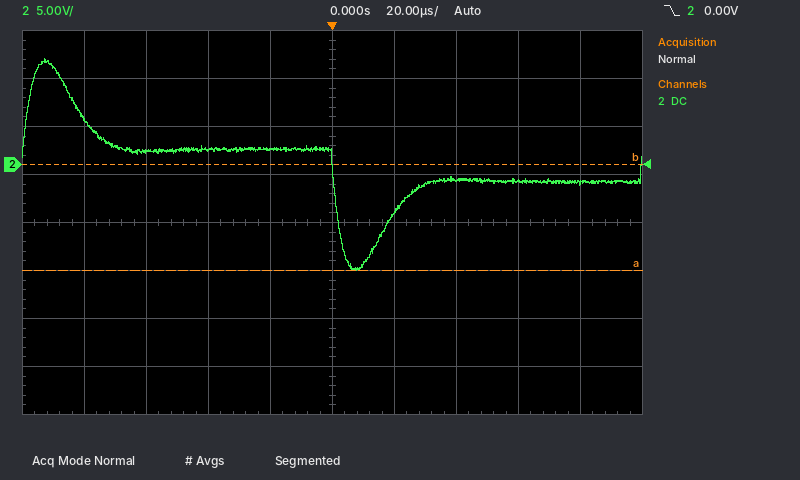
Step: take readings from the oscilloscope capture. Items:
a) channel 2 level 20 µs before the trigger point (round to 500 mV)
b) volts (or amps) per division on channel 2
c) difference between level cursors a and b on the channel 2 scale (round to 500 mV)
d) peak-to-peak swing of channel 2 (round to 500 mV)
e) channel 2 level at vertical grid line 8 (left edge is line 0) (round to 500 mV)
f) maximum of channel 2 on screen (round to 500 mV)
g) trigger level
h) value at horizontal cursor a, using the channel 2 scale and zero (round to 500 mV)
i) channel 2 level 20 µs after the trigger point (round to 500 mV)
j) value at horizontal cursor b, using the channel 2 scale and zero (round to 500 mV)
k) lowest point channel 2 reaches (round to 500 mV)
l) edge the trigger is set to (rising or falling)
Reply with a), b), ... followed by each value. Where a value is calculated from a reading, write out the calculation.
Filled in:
a) 1.5 V
b) 5 V
c) 11.0 V
d) 11.0 V − (-11.0 V) = 22.0 V
e) -1.5 V
f) 11.0 V
g) 0.00 V
h) -11.0 V
i) -5.0 V
j) 0.0 V
k) -11.0 V
l) falling
